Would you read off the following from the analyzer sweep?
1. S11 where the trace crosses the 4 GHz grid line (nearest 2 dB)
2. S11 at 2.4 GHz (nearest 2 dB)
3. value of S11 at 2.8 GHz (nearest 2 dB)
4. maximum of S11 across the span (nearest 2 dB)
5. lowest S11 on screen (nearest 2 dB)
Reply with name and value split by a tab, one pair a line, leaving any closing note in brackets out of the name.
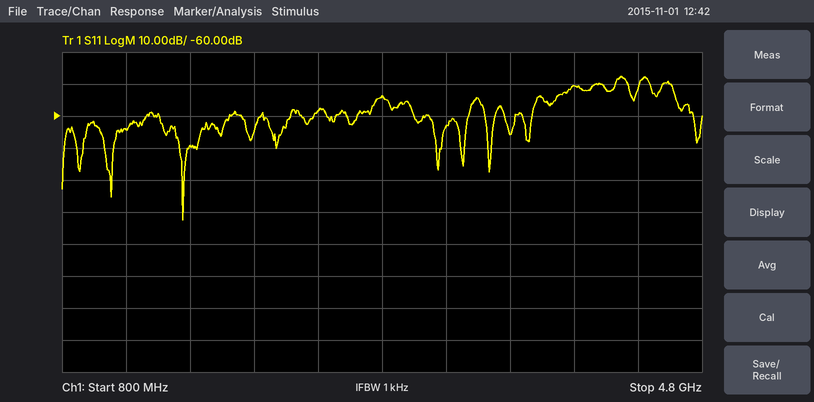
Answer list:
S11 where the trace crosses the 4 GHz grid line	-50 dB
S11 at 2.4 GHz	-58 dB
value of S11 at 2.8 GHz	-54 dB
maximum of S11 across the span	-48 dB
lowest S11 on screen	-92 dB
